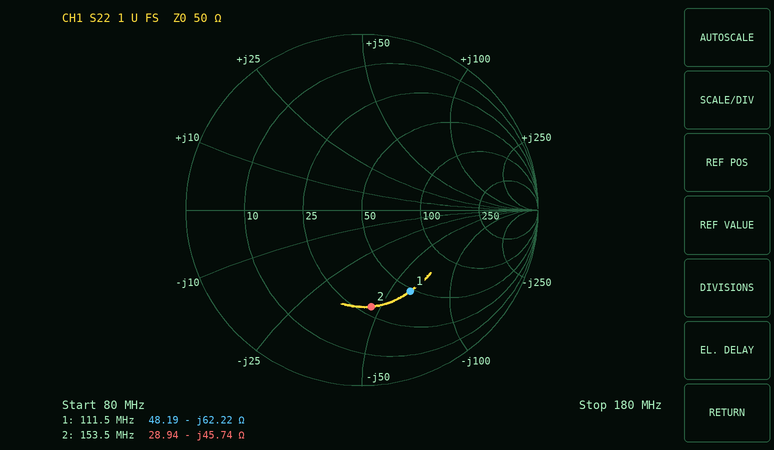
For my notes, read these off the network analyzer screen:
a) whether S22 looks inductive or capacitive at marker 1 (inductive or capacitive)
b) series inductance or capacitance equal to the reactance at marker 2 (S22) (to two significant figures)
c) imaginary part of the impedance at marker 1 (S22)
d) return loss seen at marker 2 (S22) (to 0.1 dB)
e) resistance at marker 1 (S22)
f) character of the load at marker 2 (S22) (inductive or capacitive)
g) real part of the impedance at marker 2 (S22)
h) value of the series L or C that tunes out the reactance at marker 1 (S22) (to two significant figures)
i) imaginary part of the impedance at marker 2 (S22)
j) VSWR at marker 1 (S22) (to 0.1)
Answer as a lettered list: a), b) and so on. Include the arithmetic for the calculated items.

a) capacitive
b) C = 1/(2π × 153.5 MHz × 45.74 Ω) ≈ 23 pF
c) -62.22 Ω
d) 5.2 dB
e) 48.19 Ω
f) capacitive
g) 28.94 Ω
h) L = 62.22 Ω/(2π × 111.5 MHz) ≈ 89 nH
i) -45.74 Ω
j) 3.3
